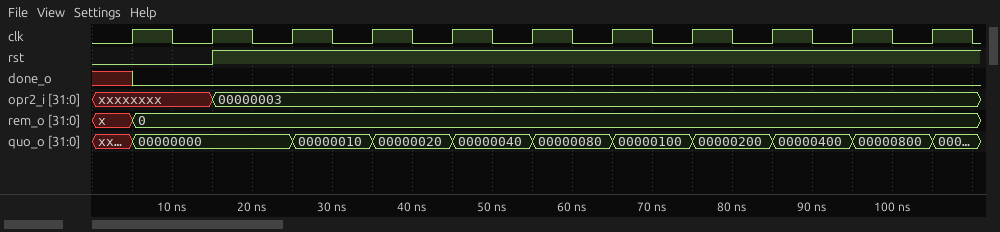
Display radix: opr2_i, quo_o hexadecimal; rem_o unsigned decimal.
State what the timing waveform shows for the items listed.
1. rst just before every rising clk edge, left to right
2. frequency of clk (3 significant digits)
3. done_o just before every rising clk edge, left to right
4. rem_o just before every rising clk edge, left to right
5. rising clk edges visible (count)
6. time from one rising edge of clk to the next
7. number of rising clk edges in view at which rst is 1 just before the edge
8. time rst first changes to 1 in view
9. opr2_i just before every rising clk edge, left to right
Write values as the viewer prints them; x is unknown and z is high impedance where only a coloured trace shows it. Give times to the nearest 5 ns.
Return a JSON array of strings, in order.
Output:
["0 0 1 1 1 1 1 1 1 1 1", "100 MHz", "x 0 0 0 0 0 0 0 0 0 0", "x, 0, 0, 0, 0, 0, 0, 0, 0, 0, 0", "11", "10 ns", "9", "15 ns", "xxxxxxxx, xxxxxxxx, 00000003, 00000003, 00000003, 00000003, 00000003, 00000003, 00000003, 00000003, 00000003"]
